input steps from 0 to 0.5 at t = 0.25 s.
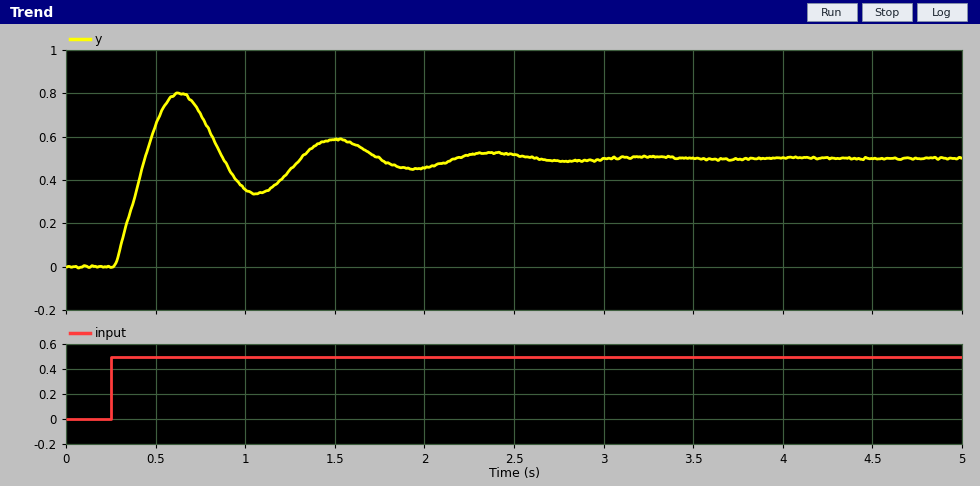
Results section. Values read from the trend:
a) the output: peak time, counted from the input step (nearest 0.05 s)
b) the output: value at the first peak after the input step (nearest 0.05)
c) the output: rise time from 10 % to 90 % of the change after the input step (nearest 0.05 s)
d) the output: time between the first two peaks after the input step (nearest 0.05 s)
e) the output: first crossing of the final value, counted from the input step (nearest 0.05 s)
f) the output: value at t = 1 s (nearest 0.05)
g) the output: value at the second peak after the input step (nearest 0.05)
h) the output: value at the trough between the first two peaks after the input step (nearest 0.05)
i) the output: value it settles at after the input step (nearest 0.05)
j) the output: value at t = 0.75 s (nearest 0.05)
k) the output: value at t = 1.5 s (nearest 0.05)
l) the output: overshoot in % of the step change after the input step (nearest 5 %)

0.40 s
0.80
0.15 s
0.85 s
0.20 s
0.35
0.60
0.35
0.50
0.70
0.60
60 %
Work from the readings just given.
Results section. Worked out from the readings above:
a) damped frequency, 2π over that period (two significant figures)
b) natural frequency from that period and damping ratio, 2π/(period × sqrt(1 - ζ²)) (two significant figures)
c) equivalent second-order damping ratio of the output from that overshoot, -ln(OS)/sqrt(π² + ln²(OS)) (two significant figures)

7.4 rad/s
7.5 rad/s
0.16
